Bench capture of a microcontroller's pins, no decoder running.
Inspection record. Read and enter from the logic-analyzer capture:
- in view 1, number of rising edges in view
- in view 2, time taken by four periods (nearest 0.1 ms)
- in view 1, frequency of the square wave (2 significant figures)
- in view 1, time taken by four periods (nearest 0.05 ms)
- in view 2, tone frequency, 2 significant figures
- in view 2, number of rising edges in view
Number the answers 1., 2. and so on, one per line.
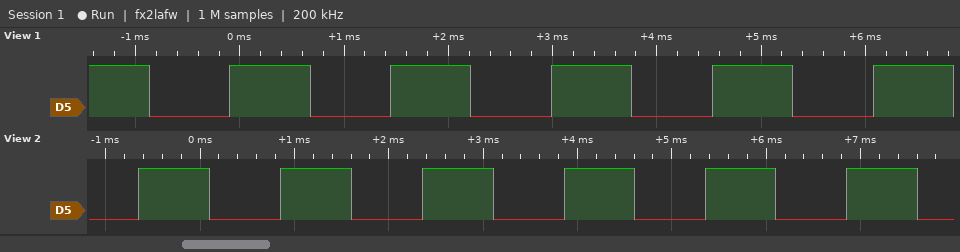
1. 5
2. 6.0 ms
3. 650 Hz
4. 6.15 ms
5. 670 Hz
6. 6
